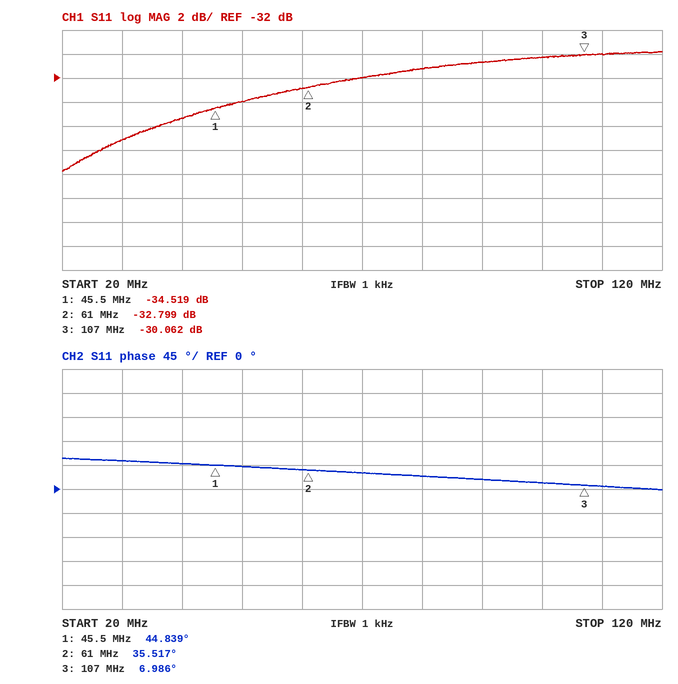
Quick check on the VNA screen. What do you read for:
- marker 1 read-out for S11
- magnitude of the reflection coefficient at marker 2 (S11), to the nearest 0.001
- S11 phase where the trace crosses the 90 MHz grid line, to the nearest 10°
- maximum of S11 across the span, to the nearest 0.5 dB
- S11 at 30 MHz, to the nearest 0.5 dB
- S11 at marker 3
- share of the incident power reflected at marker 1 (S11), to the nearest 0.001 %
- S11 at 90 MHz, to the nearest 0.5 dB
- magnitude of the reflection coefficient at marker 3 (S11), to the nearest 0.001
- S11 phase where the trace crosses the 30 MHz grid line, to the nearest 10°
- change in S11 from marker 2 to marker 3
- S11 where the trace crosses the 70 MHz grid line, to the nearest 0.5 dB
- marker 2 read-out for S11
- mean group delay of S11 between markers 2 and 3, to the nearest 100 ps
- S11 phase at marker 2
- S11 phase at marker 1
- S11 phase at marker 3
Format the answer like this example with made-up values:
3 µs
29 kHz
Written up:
-34.519 dB
0.023
20°
-30.0 dB
-37.0 dB
-30.062 dB
0.035 %
-30.5 dB
0.031
50°
2.737 dB
-32.0 dB
-32.799 dB
1.7 ns
35.517°
44.839°
6.986°
